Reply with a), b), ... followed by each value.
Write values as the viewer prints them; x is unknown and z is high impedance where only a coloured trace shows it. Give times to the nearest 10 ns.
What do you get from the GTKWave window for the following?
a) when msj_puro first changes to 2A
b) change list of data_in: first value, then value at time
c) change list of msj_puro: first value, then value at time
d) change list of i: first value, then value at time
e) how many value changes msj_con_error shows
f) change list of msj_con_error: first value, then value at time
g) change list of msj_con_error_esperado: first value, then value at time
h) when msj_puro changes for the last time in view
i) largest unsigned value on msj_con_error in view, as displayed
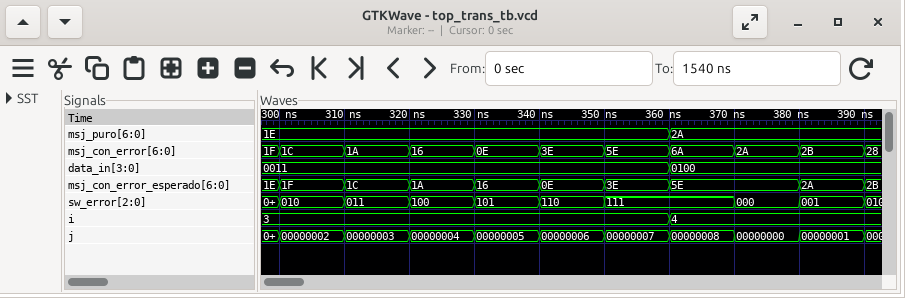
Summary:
a) 360 ns
b) 0011, 0100 at 360 ns
c) 1E, 2A at 360 ns
d) 3, 4 at 360 ns
e) 10
f) 1F, 1C at 300 ns, 1A at 310 ns, 16 at 320 ns, 0E at 330 ns, 3E at 340 ns, 5E at 350 ns, 6A at 360 ns, 2A at 370 ns, 2B at 380 ns, 28 at 390 ns
g) 1E, 1F at 300 ns, 1C at 310 ns, 1A at 320 ns, 16 at 330 ns, 0E at 340 ns, 3E at 350 ns, 5E at 360 ns, 2A at 380 ns, 2B at 390 ns
h) 360 ns
i) 6A
